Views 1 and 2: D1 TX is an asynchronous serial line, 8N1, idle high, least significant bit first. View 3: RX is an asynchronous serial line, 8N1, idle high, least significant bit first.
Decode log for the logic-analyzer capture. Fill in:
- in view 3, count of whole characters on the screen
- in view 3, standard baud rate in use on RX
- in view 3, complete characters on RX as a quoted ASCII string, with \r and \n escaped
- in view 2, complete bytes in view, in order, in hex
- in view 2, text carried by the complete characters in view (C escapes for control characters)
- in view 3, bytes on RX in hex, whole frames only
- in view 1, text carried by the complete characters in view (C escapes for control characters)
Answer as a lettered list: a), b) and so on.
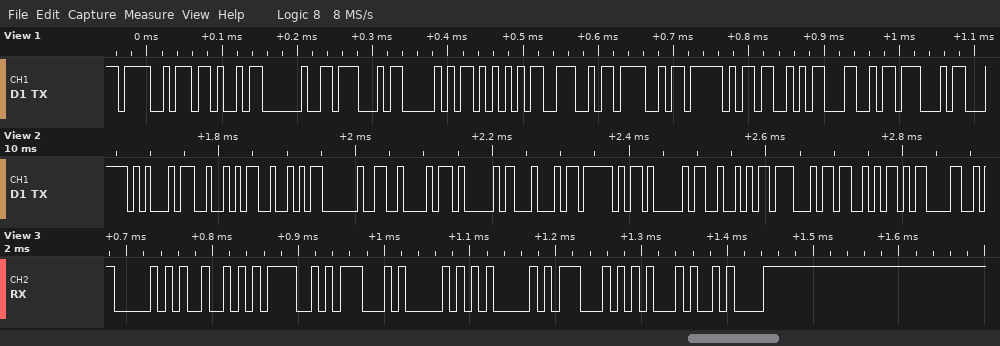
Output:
a) 9
b) 115200 baud
c) "PROGPAGE\n"
d) 45 52 52 20 42 41 44 5F 41 52 47 53 0D
e) "ERR BAD_ARGS\r"
f) 50 52 4F 47 50 41 47 45 0A
g) "OK GPUNO_SLG"
